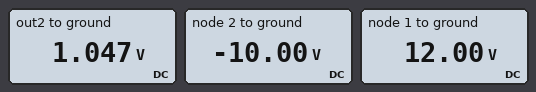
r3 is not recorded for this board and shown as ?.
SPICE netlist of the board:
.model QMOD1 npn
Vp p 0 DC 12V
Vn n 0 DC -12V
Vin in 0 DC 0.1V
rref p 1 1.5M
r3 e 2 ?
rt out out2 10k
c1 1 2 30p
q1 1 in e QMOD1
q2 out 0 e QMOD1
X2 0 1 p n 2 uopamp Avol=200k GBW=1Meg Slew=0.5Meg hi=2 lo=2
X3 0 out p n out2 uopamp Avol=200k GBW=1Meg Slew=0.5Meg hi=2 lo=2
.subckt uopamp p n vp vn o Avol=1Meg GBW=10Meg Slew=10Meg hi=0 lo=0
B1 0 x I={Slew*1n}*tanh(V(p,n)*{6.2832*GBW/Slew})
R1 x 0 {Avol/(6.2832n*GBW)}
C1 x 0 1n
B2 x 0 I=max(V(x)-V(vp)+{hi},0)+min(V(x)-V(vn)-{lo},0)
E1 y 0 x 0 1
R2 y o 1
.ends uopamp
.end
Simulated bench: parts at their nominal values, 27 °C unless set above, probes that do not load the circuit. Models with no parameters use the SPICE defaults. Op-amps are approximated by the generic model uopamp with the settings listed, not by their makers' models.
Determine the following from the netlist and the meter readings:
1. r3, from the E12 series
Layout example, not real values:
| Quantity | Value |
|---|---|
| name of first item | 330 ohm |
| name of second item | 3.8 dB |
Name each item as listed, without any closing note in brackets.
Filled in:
| Quantity | Value |
|---|---|
| r3, from the E12 series | 1.8 kΩ |
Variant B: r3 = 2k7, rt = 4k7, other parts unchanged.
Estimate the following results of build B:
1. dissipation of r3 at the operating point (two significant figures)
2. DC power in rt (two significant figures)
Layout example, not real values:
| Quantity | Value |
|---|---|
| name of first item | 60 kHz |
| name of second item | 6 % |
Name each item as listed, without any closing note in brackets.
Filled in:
| Quantity | Value |
|---|---|
| dissipation of r3 at the operating point | 32 mW |
| DC power in rt | 23 µW |
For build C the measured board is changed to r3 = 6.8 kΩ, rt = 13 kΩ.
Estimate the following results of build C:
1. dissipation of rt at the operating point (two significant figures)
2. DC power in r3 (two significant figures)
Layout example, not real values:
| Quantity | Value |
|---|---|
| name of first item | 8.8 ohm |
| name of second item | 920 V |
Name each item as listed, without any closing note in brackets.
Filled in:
| Quantity | Value |
|---|---|
| dissipation of rt at the operating point | 10 µW |
| DC power in r3 | 13 mW |
